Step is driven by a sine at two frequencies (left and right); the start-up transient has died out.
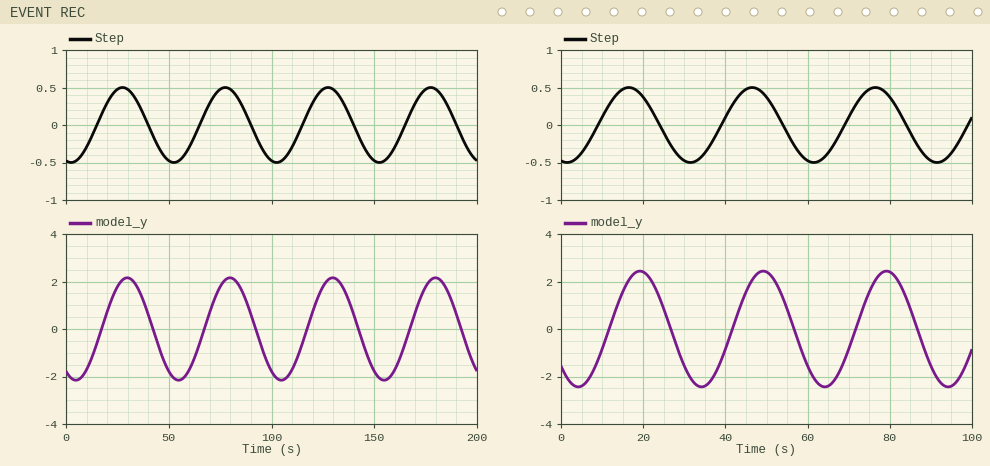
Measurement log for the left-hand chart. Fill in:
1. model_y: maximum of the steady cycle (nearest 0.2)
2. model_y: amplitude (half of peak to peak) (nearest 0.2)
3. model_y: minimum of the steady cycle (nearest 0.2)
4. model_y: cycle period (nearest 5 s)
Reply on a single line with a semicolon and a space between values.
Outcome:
2.2; 2.2; -2.2; 50 s
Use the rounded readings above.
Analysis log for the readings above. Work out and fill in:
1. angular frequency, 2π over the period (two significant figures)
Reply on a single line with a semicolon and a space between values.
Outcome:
0.13 rad/s
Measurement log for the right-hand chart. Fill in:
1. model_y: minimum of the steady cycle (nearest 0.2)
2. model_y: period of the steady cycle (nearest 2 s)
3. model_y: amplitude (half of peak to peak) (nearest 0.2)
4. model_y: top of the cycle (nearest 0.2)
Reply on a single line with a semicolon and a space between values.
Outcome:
-2.4; 30 s; 2.4; 2.4
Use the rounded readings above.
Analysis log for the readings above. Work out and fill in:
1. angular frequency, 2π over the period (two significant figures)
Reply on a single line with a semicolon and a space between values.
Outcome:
0.21 rad/s
